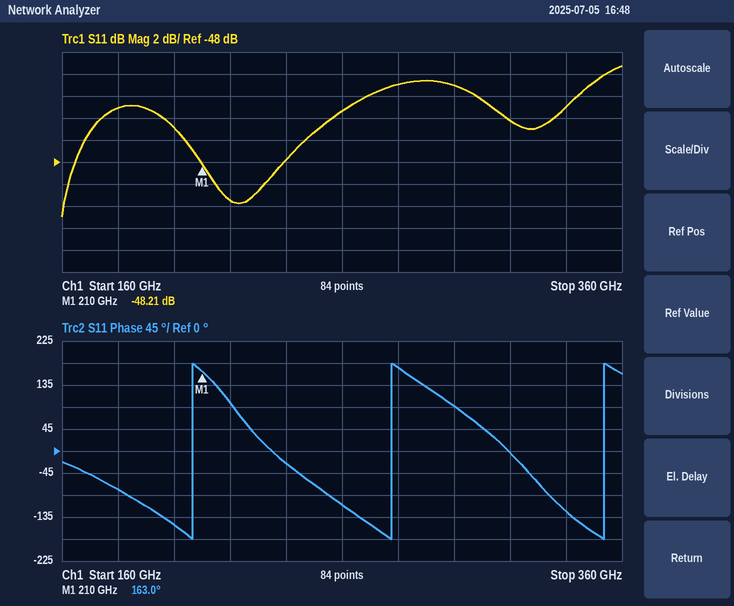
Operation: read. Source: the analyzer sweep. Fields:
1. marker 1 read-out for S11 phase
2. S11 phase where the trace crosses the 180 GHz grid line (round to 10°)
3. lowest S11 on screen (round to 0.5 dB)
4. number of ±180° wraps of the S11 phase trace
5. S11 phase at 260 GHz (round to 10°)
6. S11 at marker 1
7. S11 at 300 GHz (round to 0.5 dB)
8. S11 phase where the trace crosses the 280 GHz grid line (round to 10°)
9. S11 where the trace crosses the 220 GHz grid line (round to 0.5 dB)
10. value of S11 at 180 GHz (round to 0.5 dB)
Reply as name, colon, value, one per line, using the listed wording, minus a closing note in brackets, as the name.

marker 1 read-out for S11 phase: 163.0°
S11 phase where the trace crosses the 180 GHz grid line: -80°
lowest S11 on screen: -53.0 dB
number of ±180° wraps of the S11 phase trace: 3
S11 phase at 260 GHz: -110°
S11 at marker 1: -48.21 dB
S11 at 300 GHz: -41.0 dB
S11 phase where the trace crosses the 280 GHz grid line: 170°
S11 where the trace crosses the 220 GHz grid line: -51.5 dB
value of S11 at 180 GHz: -43.0 dB
